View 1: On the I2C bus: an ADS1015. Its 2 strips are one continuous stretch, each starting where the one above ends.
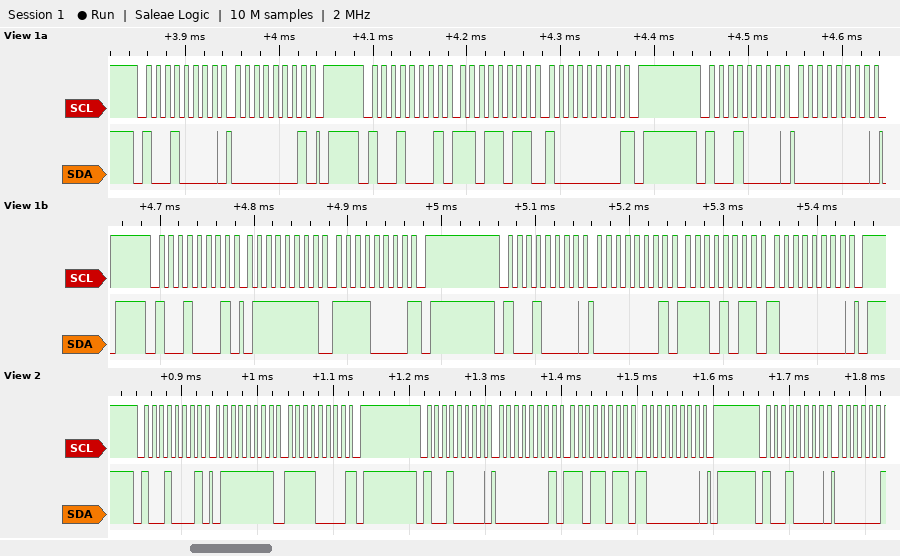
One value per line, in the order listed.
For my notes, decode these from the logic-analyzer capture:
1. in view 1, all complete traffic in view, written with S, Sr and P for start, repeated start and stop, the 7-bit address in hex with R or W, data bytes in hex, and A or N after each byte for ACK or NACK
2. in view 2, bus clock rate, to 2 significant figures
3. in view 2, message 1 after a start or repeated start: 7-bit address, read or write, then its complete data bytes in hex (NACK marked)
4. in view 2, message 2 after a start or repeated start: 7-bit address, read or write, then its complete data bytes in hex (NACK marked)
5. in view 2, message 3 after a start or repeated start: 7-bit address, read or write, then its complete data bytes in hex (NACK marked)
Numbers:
S 48W A 01 A P S 48R A DB A 80 N P S 48W A 00 A P S 48R A 7F A F0 N P S 48W A 01 A EB A 80 A P
100 kHz
0x48 read: 7F F0 NACK
0x48 write: 01 DB 80
0x48 write
